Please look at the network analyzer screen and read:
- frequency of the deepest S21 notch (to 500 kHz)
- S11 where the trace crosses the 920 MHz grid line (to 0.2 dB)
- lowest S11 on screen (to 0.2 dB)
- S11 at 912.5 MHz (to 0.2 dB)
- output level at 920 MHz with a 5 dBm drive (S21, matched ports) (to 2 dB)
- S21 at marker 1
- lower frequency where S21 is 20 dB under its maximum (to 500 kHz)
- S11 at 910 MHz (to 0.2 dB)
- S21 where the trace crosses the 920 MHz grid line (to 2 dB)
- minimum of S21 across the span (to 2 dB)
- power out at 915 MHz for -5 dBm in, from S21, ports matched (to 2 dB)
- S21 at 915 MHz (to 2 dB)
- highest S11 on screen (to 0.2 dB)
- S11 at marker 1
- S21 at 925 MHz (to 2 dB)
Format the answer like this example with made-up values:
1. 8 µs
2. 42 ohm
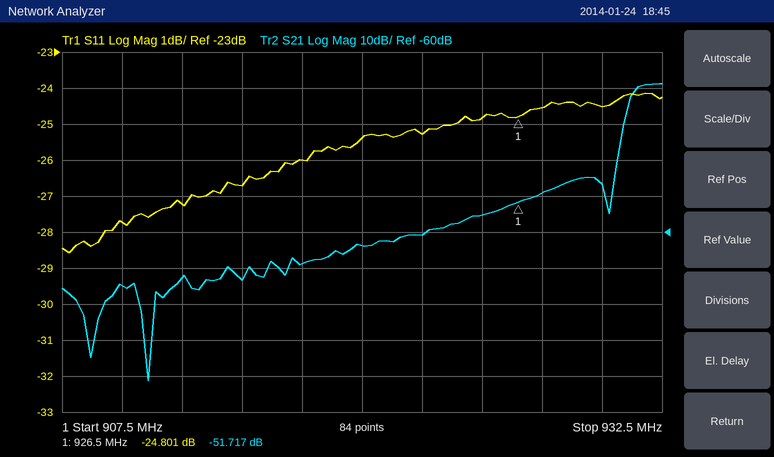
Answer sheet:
1. 911.0 MHz
2. -25.4 dB
3. -28.6 dB
4. -27.2 dB
5. -58 dBm
6. -51.717 dB
7. 930.5 MHz
8. -27.8 dB
9. -64 dB
10. -102 dB
11. -78 dBm
12. -74 dB
13. -24.2 dB
14. -24.801 dB
15. -56 dB
